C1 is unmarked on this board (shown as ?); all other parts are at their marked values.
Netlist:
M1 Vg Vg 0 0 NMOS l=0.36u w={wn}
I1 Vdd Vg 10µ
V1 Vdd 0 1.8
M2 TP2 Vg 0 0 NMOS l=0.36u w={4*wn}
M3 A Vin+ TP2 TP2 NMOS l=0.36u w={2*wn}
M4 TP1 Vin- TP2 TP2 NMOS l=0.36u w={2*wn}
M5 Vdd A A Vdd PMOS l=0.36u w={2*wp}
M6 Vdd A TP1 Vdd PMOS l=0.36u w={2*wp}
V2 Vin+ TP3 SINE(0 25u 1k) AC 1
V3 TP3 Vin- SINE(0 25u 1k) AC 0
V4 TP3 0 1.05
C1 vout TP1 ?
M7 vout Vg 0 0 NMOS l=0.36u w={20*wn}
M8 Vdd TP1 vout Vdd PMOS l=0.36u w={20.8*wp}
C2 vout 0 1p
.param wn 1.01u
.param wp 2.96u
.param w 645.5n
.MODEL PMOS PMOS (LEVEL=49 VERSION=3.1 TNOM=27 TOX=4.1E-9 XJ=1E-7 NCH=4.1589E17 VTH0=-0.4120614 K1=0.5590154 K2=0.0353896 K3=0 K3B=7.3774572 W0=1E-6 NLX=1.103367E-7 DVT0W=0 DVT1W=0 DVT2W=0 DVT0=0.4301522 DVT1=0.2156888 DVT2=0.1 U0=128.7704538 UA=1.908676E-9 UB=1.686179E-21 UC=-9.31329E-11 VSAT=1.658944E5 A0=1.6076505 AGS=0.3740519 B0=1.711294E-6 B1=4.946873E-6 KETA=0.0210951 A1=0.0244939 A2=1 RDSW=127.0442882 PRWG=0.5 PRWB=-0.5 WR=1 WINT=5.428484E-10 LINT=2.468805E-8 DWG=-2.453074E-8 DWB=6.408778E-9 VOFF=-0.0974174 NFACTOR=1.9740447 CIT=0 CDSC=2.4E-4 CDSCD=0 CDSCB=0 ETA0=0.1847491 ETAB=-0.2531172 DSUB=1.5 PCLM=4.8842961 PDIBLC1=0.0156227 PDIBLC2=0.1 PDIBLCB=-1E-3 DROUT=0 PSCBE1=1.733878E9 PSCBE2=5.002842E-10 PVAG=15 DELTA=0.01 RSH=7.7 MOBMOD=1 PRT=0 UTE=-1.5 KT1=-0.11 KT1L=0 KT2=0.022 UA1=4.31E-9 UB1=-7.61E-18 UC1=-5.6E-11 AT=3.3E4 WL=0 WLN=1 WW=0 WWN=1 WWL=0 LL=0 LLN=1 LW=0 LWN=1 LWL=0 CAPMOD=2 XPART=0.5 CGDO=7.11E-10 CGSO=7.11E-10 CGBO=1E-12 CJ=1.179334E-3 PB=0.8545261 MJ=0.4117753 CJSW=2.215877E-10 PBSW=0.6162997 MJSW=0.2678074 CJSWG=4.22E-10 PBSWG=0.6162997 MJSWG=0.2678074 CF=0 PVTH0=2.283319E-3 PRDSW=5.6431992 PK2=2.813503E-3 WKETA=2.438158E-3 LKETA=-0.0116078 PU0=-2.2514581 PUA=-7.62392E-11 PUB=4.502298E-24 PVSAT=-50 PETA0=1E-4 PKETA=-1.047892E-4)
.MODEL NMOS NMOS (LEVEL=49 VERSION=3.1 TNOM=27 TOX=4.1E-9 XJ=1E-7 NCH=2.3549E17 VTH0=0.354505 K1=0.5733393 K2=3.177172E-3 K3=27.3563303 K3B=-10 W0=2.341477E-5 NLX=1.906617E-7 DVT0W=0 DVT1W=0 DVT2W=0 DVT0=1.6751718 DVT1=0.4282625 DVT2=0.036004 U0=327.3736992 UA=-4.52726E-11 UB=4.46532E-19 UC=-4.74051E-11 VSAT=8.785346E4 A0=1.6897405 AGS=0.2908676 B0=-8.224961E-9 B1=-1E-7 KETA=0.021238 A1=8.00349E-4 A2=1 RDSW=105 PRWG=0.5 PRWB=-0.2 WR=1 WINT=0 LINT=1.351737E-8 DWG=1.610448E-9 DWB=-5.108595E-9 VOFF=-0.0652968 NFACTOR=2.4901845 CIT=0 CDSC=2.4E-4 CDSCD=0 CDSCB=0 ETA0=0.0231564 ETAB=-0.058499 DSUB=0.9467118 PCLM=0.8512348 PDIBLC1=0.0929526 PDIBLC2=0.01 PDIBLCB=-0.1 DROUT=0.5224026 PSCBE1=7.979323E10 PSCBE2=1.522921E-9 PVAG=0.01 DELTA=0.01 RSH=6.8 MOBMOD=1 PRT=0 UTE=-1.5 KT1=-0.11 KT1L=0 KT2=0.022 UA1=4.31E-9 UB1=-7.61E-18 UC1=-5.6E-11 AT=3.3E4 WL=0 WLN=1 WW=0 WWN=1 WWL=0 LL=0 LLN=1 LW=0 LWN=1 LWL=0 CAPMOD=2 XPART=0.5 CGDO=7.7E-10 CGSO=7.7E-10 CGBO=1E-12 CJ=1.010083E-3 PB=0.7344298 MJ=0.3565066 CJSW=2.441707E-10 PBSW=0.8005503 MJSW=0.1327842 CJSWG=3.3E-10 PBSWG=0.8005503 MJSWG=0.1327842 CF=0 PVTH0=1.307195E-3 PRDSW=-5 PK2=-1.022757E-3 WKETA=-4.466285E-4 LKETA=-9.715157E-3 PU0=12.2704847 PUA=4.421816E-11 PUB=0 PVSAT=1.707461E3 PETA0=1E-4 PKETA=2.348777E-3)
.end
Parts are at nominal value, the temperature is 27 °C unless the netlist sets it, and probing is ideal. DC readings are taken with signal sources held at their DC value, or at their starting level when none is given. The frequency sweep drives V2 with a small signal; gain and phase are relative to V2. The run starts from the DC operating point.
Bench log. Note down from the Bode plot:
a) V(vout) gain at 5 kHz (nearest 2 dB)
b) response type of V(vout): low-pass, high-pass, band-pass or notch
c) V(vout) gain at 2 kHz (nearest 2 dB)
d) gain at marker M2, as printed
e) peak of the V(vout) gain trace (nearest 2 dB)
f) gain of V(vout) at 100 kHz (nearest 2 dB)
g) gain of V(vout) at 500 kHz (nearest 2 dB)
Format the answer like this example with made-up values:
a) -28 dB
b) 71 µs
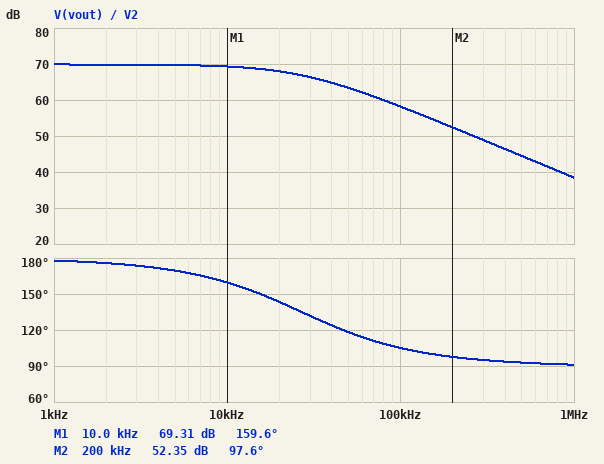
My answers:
a) 70 dB
b) low-pass
c) 70 dB
d) 52.35 dB
e) 70 dB
f) 58 dB
g) 44 dB
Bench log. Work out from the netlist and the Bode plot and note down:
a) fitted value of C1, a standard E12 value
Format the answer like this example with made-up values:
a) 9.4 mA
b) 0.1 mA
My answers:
a) 390 fF
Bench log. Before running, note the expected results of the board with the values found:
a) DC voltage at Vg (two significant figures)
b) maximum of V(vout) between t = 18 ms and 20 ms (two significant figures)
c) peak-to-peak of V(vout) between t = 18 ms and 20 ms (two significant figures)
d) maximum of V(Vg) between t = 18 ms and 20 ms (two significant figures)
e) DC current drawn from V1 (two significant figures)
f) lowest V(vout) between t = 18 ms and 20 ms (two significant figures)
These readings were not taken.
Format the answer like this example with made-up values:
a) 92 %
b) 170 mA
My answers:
a) 650 mV
b) 1.1 V
c) 310 mV
d) 650 mV
e) 250 µA
f) 760 mV
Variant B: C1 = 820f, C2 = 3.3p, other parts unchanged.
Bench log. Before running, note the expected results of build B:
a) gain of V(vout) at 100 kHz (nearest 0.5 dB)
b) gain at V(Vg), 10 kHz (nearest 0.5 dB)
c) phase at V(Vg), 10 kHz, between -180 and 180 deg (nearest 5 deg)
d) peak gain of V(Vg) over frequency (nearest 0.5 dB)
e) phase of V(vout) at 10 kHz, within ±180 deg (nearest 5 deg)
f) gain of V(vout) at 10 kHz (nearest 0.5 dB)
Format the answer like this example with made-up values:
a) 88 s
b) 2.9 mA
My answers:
a) 52.5 dB
b) -34.0 dB
c) -125 deg
d) -29.5 dB
e) 145 deg
f) 68.0 dB
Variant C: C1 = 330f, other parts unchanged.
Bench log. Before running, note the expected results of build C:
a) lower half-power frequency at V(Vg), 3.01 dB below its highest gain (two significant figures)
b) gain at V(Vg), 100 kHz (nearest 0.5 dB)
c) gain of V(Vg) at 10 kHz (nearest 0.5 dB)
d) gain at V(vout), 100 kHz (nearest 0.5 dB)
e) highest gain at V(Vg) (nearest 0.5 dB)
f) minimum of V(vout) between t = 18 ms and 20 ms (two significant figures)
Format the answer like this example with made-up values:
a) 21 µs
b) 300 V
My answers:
a) 31 kHz
b) -23.0 dB
c) -32.5 dB
d) 59.5 dB
e) -22.5 dB
f) 760 mV
